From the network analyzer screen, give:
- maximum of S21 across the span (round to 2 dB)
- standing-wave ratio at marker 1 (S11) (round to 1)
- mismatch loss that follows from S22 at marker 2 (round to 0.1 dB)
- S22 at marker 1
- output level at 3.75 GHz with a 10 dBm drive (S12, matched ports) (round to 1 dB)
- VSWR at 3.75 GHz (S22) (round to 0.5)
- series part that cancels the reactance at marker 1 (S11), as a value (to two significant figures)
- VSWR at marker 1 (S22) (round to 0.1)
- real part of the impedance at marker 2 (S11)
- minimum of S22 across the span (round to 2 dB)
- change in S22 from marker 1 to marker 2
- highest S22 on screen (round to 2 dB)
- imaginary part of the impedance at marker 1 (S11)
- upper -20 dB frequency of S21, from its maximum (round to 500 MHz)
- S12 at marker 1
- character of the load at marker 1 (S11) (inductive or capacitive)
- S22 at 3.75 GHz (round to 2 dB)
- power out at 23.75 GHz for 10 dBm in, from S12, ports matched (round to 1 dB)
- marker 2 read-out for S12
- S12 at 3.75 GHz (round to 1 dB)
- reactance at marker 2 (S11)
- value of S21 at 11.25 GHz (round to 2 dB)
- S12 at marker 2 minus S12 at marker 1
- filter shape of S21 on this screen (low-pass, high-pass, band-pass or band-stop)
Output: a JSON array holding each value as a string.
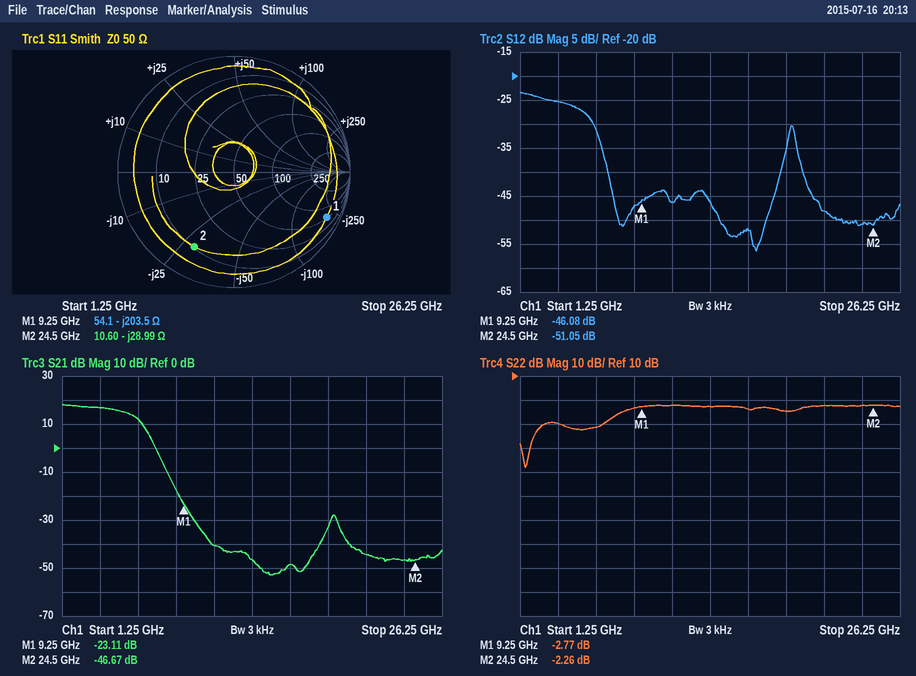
["18 dB", "17", "3.9 dB", "-2.77 dB", "-15 dBm", "2.0", "3.5 nH", "6.3", "10.60 Ω", "-28 dB", "0.51 dB", "-2 dB", "-203.5 Ω", "7.5 GHz", "-46.08 dB", "capacitive", "-10 dB", "-41 dBm", "-51.05 dB", "-25 dB", "-28.99 Ω", "-40 dB", "-4.97 dB", "low-pass"]
